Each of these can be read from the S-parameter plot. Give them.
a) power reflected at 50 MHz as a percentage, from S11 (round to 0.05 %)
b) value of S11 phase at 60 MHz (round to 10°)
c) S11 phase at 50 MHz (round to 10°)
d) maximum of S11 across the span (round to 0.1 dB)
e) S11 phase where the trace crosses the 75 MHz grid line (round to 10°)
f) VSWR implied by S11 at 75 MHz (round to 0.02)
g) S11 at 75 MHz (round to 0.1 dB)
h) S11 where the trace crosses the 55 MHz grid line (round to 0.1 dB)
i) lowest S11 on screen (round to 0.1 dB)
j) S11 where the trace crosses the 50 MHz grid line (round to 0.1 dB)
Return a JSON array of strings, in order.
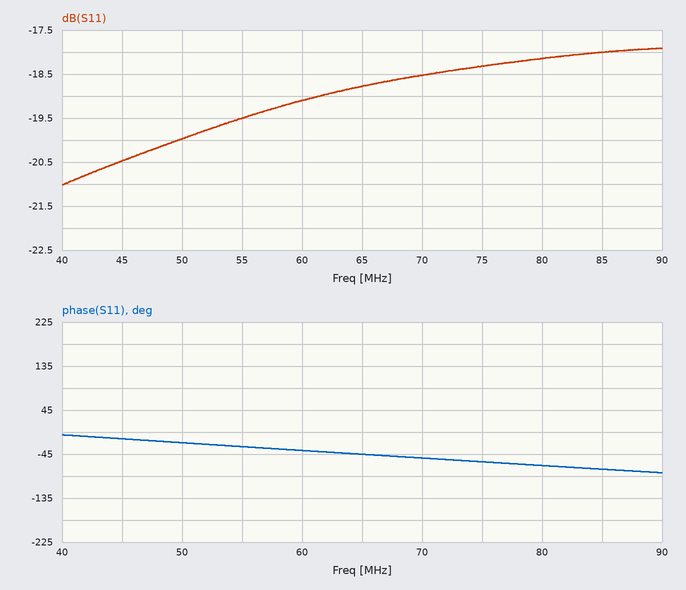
["1.00 %", "-40°", "-20°", "-17.9 dB", "-60°", "1.28", "-18.3 dB", "-19.5 dB", "-21.0 dB", "-20.0 dB"]
